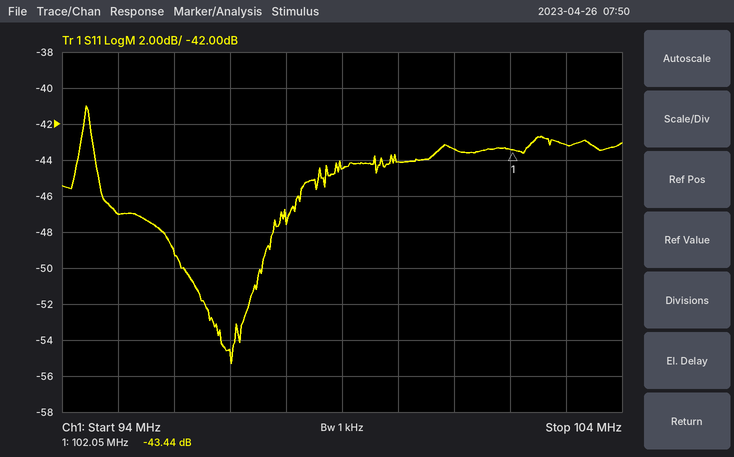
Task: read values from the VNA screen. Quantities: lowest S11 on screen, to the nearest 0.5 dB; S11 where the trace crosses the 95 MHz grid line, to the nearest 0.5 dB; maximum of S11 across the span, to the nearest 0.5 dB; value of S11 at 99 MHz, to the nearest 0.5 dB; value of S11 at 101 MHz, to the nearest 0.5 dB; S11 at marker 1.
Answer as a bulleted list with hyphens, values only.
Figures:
- -55.5 dB
- -47.0 dB
- -41.0 dB
- -44.5 dB
- -43.5 dB
- -43.44 dB
